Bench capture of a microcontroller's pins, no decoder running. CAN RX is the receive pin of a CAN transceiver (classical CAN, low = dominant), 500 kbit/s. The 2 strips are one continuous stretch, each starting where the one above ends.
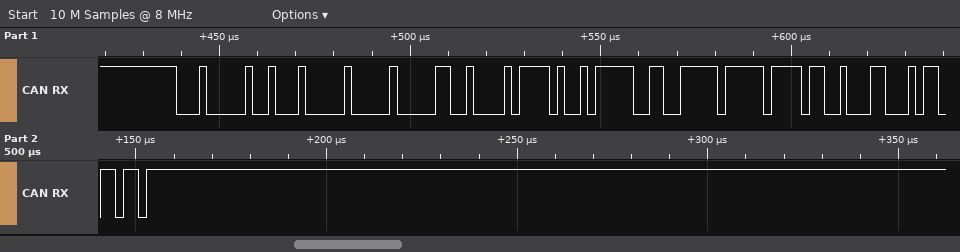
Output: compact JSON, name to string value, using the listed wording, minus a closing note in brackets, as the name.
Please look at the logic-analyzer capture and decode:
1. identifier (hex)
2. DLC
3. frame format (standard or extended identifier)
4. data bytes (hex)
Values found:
{"identifier": "0x101", "DLC": "8", "frame format": "standard", "data bytes": "00 09 0B D2 FB 3F FF 64"}
